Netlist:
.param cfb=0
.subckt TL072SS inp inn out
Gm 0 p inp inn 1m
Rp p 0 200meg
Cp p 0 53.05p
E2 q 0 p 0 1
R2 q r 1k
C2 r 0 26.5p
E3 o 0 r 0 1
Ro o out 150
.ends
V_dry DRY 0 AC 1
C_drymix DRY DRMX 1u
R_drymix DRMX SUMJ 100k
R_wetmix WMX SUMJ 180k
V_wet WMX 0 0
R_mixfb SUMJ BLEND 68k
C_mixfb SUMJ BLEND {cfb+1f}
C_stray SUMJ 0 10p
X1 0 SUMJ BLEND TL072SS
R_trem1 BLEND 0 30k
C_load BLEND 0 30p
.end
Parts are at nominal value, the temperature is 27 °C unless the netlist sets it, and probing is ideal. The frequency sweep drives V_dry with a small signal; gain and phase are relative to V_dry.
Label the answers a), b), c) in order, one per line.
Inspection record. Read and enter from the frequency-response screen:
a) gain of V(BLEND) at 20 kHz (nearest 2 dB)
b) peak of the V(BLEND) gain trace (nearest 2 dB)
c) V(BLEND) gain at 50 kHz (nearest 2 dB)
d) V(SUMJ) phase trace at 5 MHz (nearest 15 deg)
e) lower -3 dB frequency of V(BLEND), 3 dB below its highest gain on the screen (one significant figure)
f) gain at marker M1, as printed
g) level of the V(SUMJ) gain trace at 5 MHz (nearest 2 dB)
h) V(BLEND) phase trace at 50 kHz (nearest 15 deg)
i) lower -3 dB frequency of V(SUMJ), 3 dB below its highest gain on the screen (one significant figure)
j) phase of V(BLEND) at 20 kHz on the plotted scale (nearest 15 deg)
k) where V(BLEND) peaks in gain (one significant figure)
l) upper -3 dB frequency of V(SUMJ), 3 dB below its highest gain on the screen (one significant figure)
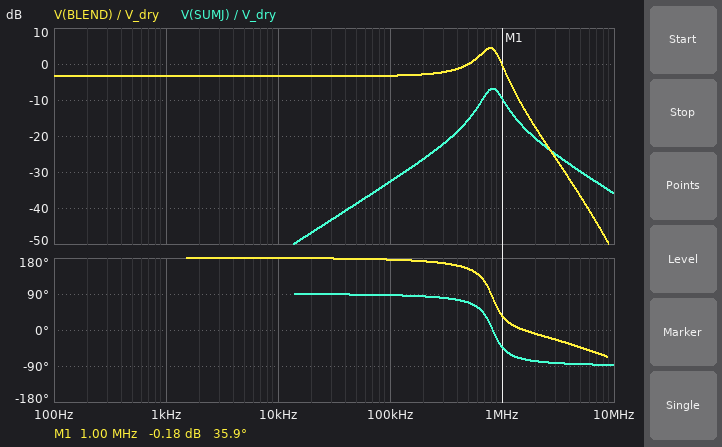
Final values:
a) -4 dB
b) 4 dB
c) -4 dB
d) -90 deg
e) 600 kHz
f) -0.18 dB
g) -30 dB
h) 180 deg
i) 700 kHz
j) 180 deg
k) 800 kHz
l) 1 MHz
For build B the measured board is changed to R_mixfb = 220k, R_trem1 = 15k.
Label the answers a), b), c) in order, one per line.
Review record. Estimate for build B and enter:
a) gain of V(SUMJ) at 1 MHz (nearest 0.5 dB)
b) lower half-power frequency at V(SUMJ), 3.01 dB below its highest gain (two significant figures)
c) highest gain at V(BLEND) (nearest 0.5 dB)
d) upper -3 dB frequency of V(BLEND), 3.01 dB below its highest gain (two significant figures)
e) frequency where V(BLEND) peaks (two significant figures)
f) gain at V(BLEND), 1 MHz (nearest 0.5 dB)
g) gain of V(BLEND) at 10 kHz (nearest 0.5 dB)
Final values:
a) -14.5 dB
b) 340 kHz
c) 11.5 dB
d) 540 kHz
e) 420 kHz
f) -5.0 dB
g) 7.0 dB
